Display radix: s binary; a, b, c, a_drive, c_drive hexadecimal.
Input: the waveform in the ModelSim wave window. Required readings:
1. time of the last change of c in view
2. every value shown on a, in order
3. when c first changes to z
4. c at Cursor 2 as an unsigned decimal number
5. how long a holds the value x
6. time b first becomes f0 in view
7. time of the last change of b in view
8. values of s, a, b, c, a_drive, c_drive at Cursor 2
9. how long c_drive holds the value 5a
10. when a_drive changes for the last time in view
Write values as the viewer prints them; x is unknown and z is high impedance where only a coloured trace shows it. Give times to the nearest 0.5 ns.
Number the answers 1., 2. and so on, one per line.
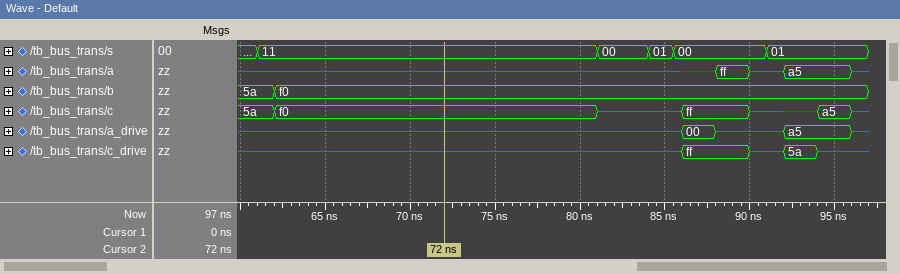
1. 96 ns
2. z, x, ff, z, a5, z
3. 81 ns
4. 240
5. 2 ns
6. 62 ns
7. 62 ns
8. s=11, a=z, b=f0, c=f0, a_drive=z, c_drive=z
9. 2 ns
10. 96 ns
